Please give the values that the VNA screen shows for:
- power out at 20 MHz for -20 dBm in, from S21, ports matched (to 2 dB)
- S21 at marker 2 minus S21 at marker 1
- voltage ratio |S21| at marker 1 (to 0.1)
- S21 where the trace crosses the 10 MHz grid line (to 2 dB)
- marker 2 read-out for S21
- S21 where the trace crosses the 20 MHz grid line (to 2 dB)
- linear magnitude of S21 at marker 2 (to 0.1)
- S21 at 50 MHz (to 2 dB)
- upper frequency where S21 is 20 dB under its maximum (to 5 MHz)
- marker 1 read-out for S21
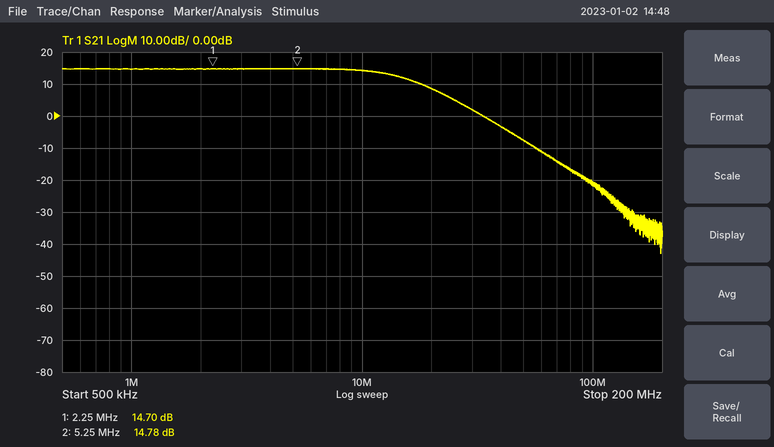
-12 dBm
0.08 dB
5.4
14 dB
14.78 dB
8 dB
5.5
-8 dB
45 MHz
14.70 dB
